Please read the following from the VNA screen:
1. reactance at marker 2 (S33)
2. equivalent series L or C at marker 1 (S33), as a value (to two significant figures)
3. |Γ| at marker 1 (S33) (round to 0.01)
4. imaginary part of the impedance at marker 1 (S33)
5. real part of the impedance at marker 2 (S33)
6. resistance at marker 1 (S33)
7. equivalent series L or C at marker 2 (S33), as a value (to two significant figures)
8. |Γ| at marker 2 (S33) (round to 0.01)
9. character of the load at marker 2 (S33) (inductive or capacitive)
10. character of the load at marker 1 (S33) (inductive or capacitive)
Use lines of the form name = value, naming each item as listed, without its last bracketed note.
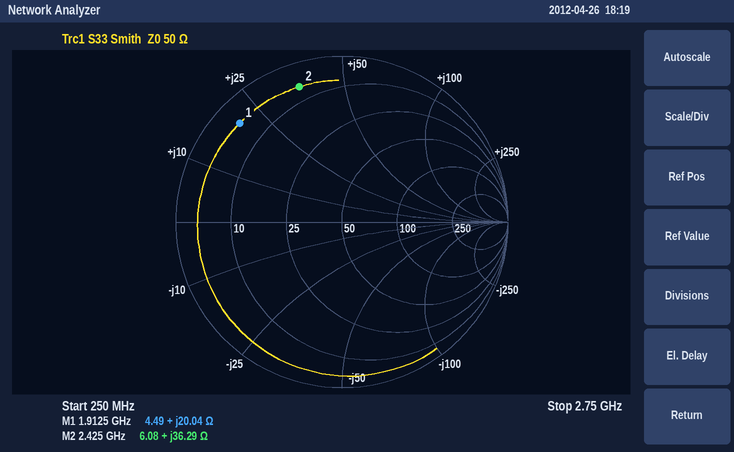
reactance at marker 2 = +36.29 Ω
equivalent series L or C at marker 1 (S33), as a value = 1.7 nH
|Γ| at marker 1 (S33) = 0.86
imaginary part of the impedance at marker 1 = +20.04 Ω
real part of the impedance at marker 2 = 6.08 Ω
resistance at marker 1 = 4.49 Ω
equivalent series L or C at marker 2 (S33), as a value = 2.4 nH
|Γ| at marker 2 (S33) = 0.85
character of the load at marker 2 (S33) = inductive
character of the load at marker 1 (S33) = inductive
